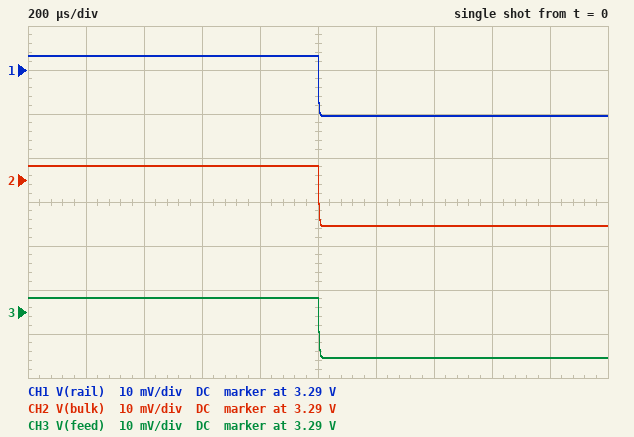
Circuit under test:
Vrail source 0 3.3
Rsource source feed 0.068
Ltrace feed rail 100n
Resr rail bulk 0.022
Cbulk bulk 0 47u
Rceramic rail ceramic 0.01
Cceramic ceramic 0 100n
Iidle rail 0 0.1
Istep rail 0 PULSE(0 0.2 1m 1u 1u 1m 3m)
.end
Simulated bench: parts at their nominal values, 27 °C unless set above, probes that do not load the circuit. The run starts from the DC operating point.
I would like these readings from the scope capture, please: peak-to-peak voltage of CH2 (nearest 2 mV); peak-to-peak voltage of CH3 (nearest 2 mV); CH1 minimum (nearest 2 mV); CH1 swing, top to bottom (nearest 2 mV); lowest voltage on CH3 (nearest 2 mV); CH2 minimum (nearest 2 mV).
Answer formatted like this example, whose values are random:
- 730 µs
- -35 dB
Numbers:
- 14 mV
- 14 mV
- 3.280 V
- 14 mV
- 3.280 V
- 3.280 V
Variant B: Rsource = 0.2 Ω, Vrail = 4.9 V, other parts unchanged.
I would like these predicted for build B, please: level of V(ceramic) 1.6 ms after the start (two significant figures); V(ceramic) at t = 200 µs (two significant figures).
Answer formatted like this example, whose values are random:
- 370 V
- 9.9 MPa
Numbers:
- 4.8 V
- 4.9 V
